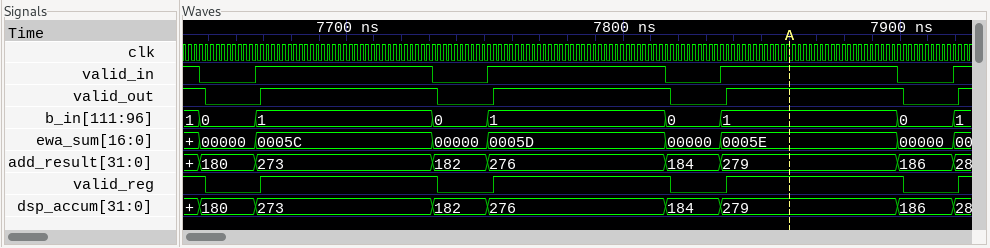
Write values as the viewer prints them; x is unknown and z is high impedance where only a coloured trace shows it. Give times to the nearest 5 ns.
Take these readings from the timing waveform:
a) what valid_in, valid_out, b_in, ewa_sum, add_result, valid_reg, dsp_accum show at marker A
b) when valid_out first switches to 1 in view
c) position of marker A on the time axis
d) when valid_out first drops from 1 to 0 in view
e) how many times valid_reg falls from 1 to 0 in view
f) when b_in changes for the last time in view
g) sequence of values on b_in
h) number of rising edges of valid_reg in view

valid_in=1, valid_out=1, b_in=1, ewa_sum=0005E, add_result=279, valid_reg=1, dsp_accum=279
7670 ns
7860 ns
7650 ns
4
7920 ns
1, 0, 1, 0, 1, 0, 1, 0, 1
4
